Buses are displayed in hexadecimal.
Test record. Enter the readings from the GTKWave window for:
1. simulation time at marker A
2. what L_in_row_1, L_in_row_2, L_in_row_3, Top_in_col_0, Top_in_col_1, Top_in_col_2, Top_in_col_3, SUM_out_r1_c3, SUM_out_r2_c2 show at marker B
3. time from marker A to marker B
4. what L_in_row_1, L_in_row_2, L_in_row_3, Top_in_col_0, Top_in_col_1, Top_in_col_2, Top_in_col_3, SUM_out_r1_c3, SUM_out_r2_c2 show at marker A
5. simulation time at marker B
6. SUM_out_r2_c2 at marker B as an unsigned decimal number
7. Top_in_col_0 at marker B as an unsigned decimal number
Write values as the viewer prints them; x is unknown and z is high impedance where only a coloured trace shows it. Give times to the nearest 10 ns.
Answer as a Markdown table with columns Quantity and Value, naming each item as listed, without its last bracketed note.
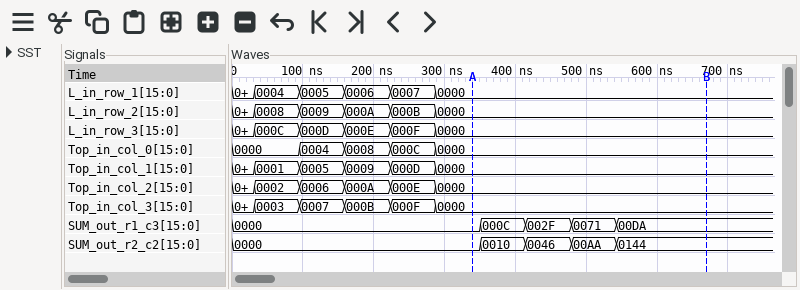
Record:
| Quantity | Value |
|---|---|
| simulation time at marker A | 340 ns |
| what L_in_row_1, L_in_row_2, L_in_row_3, Top_in_col_0, Top_in_col_1, Top_in_col_2, Top_in_col_3, SUM_out_r1_c3, SUM_out_r2_c2 show at marker B | L_in_row_1=0000, L_in_row_2=0000, L_in_row_3=0000, Top_in_col_0=0000, Top_in_col_1=0000, Top_in_col_2=0000, Top_in_col_3=0000, SUM_out_r1_c3=00DA, SUM_out_r2_c2=0144 |
| time from marker A to marker B | 330 ns |
| what L_in_row_1, L_in_row_2, L_in_row_3, Top_in_col_0, Top_in_col_1, Top_in_col_2, Top_in_col_3, SUM_out_r1_c3, SUM_out_r2_c2 show at marker A | L_in_row_1=0000, L_in_row_2=0000, L_in_row_3=0000, Top_in_col_0=0000, Top_in_col_1=0000, Top_in_col_2=0000, Top_in_col_3=0000, SUM_out_r1_c3=0000, SUM_out_r2_c2=0000 |
| simulation time at marker B | 670 ns |
| SUM_out_r2_c2 at marker B as an unsigned decimal number | 324 |
| Top_in_col_0 at marker B as an unsigned decimal number | 0 |
